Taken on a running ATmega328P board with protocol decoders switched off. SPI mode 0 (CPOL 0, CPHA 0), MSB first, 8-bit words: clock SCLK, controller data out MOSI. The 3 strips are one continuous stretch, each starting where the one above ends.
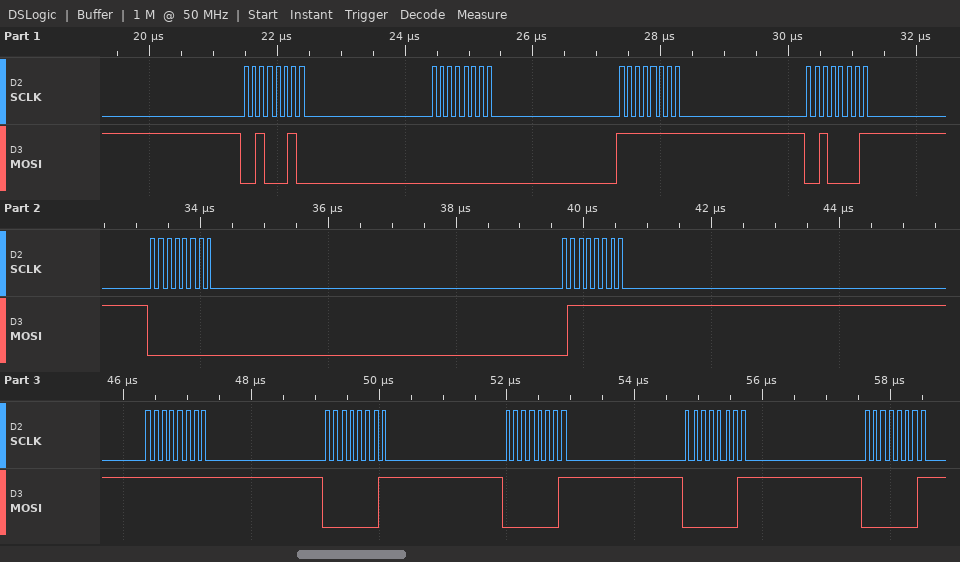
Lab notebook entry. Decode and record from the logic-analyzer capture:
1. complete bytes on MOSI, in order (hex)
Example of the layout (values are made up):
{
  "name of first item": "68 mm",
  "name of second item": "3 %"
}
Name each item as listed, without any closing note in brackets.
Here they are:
{
  "complete bytes on MOSI, in order": "22 00 FF 21 00 7F FF 01 01 01 01"
}
